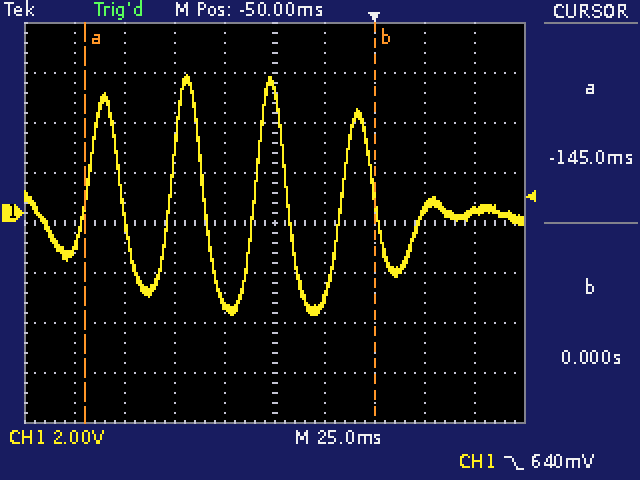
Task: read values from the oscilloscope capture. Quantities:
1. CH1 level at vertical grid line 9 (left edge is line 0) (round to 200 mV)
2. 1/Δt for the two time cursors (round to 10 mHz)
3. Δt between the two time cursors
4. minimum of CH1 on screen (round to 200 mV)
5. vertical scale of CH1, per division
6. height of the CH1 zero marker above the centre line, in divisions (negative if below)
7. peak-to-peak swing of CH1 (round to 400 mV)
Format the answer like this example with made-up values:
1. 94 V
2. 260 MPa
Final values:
1. 0.0 V
2. 6.90 Hz
3. 145.0 ms
4. -4.0 V
5. 2 V
6. +0.2 div
7. 9.6 V
